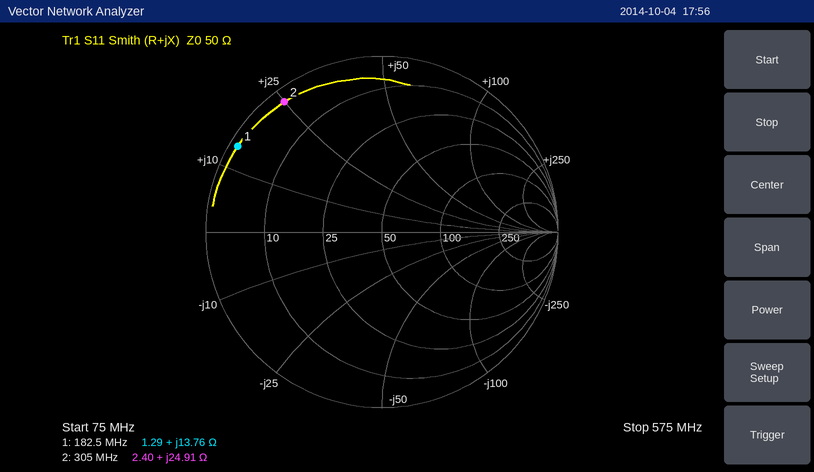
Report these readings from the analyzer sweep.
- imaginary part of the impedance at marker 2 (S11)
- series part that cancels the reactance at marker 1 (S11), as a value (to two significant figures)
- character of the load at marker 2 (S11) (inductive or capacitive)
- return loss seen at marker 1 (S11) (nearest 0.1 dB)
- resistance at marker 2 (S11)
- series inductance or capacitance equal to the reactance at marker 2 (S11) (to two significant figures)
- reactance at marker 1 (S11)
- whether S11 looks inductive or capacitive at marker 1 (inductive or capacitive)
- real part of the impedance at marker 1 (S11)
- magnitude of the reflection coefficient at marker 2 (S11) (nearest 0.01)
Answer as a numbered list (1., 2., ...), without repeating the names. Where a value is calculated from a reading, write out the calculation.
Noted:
1. +24.91 Ω
2. C = 1/(2π × 182.5 MHz × 13.76 Ω) ≈ 63 pF
3. inductive
4. 0.4 dB
5. 2.40 Ω
6. L = 24.91 Ω/(2π × 305 MHz) ≈ 13 nH
7. +13.76 Ω
8. inductive
9. 1.29 Ω
10. 0.93
